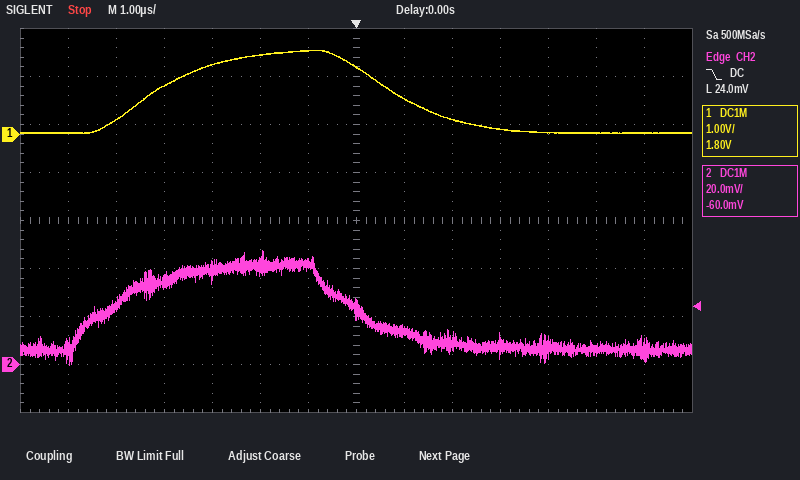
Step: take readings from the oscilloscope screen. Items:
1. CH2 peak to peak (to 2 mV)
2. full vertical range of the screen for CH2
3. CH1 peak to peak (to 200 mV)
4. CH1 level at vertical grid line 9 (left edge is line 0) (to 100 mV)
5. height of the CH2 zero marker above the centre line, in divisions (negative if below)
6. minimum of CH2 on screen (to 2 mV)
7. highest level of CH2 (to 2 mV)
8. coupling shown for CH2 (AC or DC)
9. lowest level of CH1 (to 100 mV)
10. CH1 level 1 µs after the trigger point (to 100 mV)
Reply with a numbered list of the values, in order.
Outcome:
1. 48 mV
2. 160 mV
3. 1.8 V
4. 300 mV
5. -3.0 div
6. 0 mV
7. 48 mV
8. DC
9. 0.0 V
10. 700 mV
